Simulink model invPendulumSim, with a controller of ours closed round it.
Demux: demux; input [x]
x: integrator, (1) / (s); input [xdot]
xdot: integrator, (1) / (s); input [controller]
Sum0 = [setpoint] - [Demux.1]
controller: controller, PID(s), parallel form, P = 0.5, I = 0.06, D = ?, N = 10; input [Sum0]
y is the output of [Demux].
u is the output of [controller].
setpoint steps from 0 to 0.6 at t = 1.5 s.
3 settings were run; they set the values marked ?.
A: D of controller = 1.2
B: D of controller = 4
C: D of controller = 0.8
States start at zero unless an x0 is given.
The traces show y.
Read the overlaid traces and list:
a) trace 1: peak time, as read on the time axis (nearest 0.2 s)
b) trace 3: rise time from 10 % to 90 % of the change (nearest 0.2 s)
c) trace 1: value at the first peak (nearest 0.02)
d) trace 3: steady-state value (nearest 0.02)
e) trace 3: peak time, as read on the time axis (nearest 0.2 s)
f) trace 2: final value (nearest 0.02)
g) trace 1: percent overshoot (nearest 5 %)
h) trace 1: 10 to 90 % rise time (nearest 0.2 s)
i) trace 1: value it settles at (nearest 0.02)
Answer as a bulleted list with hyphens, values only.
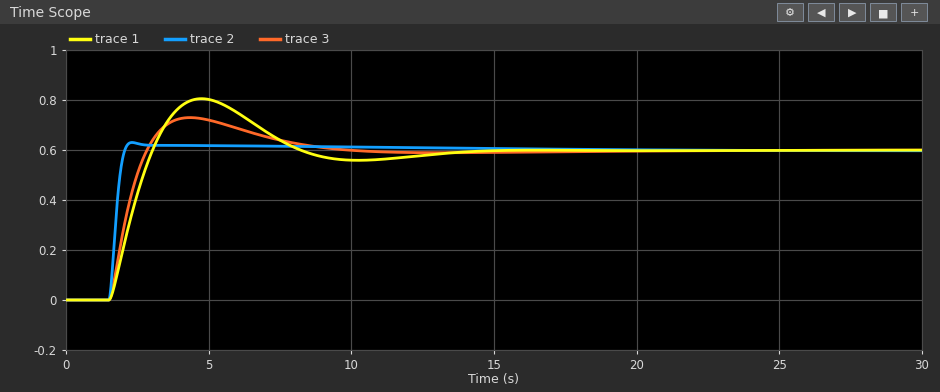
- 4.8 s
- 1.0 s
- 0.80
- 0.60
- 4.4 s
- 0.60
- 35 %
- 1.2 s
- 0.60
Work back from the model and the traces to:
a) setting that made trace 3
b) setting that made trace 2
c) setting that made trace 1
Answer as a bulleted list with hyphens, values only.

- A
- B
- C
